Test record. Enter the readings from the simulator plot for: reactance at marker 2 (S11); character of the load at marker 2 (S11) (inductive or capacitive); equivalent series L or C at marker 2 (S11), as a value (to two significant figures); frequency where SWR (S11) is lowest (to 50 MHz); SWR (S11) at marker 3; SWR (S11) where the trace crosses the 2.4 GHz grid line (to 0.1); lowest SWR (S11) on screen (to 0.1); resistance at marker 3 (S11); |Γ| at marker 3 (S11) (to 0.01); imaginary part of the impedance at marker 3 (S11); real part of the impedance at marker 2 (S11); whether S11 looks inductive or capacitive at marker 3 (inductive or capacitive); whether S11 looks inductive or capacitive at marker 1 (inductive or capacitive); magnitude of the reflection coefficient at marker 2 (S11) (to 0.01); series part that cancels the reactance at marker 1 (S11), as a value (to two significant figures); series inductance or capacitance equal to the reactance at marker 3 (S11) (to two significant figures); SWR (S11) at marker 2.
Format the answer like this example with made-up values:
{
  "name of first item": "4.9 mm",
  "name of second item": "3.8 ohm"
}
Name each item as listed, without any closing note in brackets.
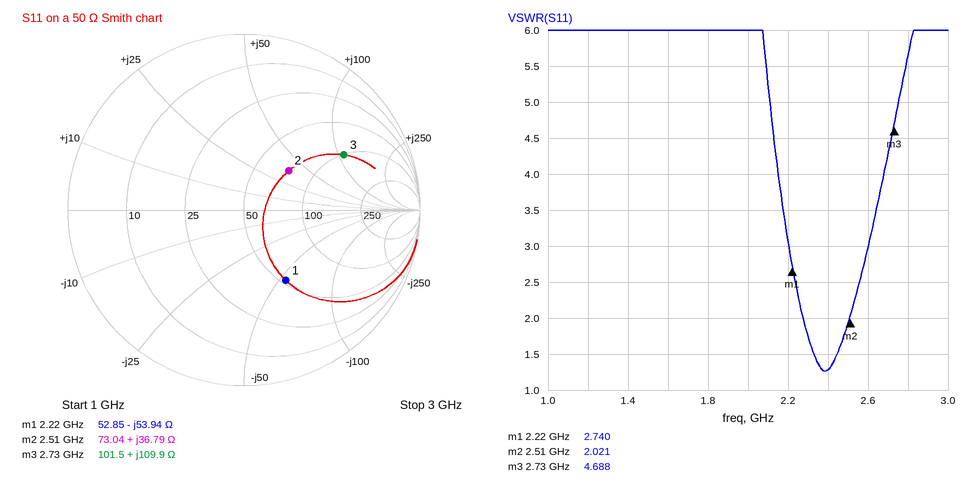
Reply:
{
  "reactance at marker 2": "+36.79 Ω",
  "character of the load at marker 2 (S11)": "inductive",
  "equivalent series L or C at marker 2 (S11), as a value": "2.3 nH",
  "frequency where SWR (S11) is lowest": "2.40 GHz",
  "SWR (S11) at marker 3": "4.688",
  "SWR (S11) where the trace crosses the 2.4 GHz grid line": "1.3",
  "lowest SWR (S11) on screen": "1.3",
  "resistance at marker 3": "101.5 Ω",
  "|Γ| at marker 3 (S11)": "0.65",
  "imaginary part of the impedance at marker 3": "+109.9 Ω",
  "real part of the impedance at marker 2": "73.04 Ω",
  "whether S11 looks inductive or capacitive at marker 3": "inductive",
  "whether S11 looks inductive or capacitive at marker 1": "capacitive",
  "magnitude of the reflection coefficient at marker 2 (S11)": "0.34",
  "series part that cancels the reactance at marker 1 (S11), as a value": "3.9 nH",
  "series inductance or capacitance equal to the reactance at marker 3 (S11)": "6.4 nH",
  "SWR (S11) at marker 2": "2.021"
}
